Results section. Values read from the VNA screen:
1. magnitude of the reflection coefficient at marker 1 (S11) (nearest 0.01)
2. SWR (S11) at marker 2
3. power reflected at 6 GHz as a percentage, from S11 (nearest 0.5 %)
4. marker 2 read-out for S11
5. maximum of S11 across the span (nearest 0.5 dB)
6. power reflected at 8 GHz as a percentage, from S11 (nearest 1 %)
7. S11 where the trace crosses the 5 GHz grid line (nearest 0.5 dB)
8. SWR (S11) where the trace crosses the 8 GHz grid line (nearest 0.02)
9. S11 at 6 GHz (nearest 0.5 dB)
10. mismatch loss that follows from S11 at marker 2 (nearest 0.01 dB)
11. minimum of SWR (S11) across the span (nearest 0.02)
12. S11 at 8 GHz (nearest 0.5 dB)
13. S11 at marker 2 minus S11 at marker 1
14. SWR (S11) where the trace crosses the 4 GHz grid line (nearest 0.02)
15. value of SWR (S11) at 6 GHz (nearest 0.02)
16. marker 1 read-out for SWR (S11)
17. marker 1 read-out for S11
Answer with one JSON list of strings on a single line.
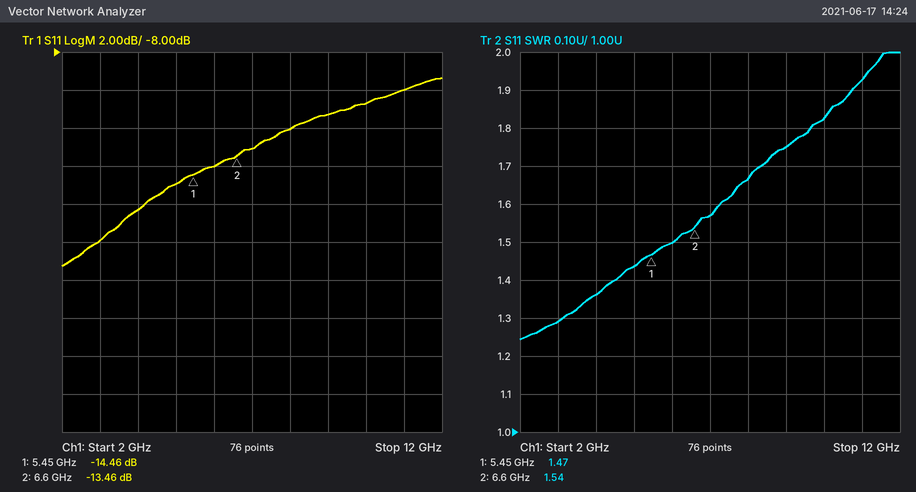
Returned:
["0.19", "1.54", "4.0 %", "-13.46 dB", "-9.5 dB", "6 %", "-15.0 dB", "1.66", "-14.0 dB", "0.20 dB", "1.24", "-12.0 dB", "1.00 dB", "1.36", "1.50", "1.47", "-14.46 dB"]
